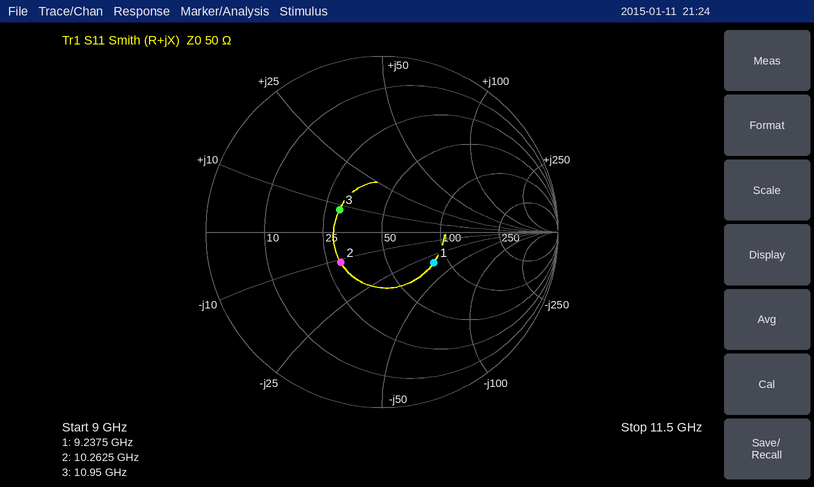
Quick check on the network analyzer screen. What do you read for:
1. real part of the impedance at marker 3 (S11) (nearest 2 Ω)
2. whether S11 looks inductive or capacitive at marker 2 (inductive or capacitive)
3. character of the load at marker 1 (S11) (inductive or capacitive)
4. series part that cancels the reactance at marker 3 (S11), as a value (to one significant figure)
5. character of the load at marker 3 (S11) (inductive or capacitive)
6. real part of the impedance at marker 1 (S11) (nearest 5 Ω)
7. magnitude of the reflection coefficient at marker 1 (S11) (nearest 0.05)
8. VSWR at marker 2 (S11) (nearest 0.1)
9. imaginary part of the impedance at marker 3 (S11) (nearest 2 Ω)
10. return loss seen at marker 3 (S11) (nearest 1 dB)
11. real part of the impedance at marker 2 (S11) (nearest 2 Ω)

30 Ω
capacitive
capacitive
2 pF
inductive
85 Ω
0.35
1.8
+8 Ω
11 dB
30 Ω
